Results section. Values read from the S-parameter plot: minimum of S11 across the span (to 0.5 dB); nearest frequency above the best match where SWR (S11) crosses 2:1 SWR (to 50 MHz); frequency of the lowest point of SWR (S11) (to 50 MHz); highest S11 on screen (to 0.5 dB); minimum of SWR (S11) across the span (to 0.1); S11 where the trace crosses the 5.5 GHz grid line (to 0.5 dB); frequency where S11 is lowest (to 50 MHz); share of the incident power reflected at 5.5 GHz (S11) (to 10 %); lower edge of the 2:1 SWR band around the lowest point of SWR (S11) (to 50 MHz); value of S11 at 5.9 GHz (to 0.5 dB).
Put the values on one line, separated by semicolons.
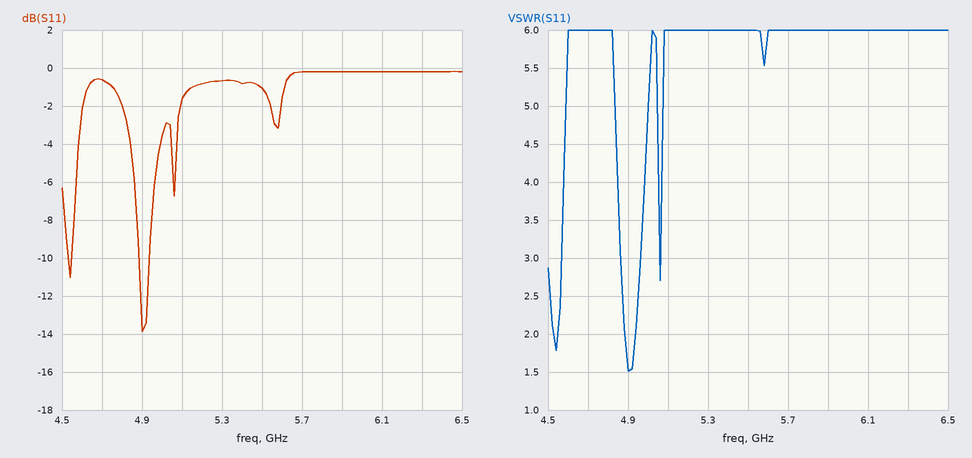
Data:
-14.0 dB; 4.95 GHz; 4.90 GHz; 0.0 dB; 1.5; -1.0 dB; 4.90 GHz; 80 %; 4.90 GHz; 0.0 dB
